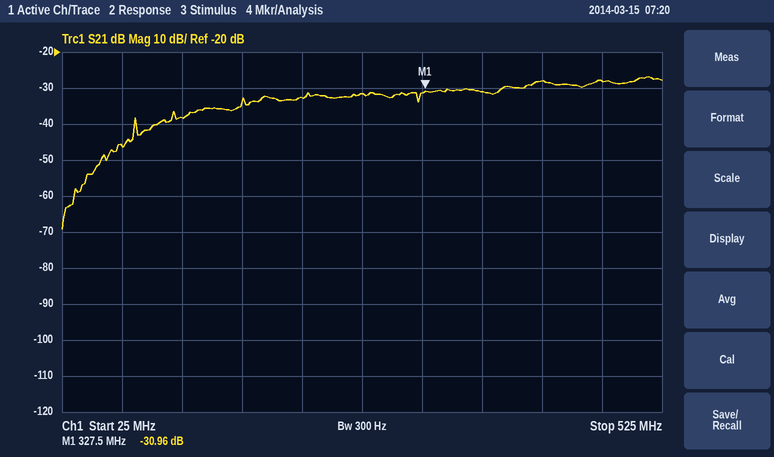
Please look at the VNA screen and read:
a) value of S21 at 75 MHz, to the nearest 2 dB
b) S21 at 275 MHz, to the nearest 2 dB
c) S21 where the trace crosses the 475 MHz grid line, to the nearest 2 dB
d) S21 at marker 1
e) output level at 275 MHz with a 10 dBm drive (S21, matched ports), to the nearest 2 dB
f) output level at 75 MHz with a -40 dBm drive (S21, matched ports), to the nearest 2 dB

-46 dB
-32 dB
-28 dB
-30.96 dB
-22 dBm
-86 dBm
